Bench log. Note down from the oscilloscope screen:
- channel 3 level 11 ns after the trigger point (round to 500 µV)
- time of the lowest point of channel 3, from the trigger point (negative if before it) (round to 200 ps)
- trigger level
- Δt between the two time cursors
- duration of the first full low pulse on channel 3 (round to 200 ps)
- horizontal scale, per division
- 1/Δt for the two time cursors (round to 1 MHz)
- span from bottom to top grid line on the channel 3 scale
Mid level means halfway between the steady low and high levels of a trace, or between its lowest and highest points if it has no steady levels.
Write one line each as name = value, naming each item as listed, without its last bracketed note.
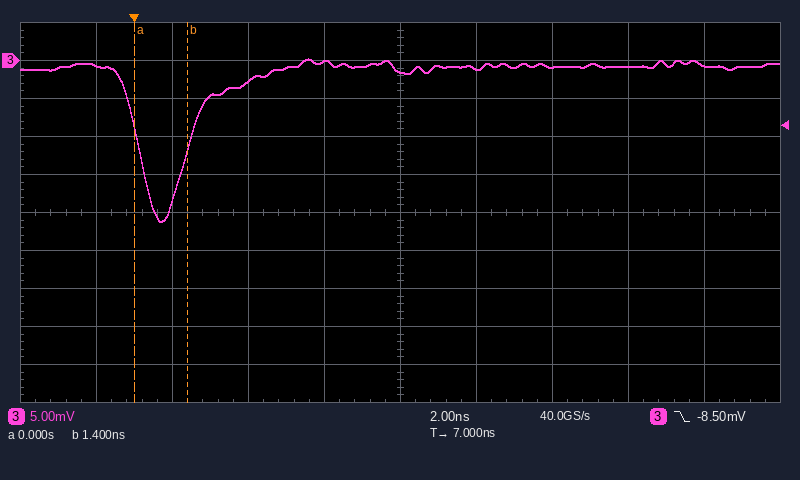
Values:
channel 3 level 11 ns after the trigger point = -1.0 mV
time of the lowest point of channel 3, from the trigger point (negative if before it) = +800 ps
trigger level = -8.50 mV
Δt between the two time cursors = 1.4 ns
duration of the first full low pulse on channel 3 = 1.4 ns
horizontal scale, per division = 2 ns
1/Δt for the two time cursors = 714 MHz
span from bottom to top grid line on the channel 3 scale = 50 mV
